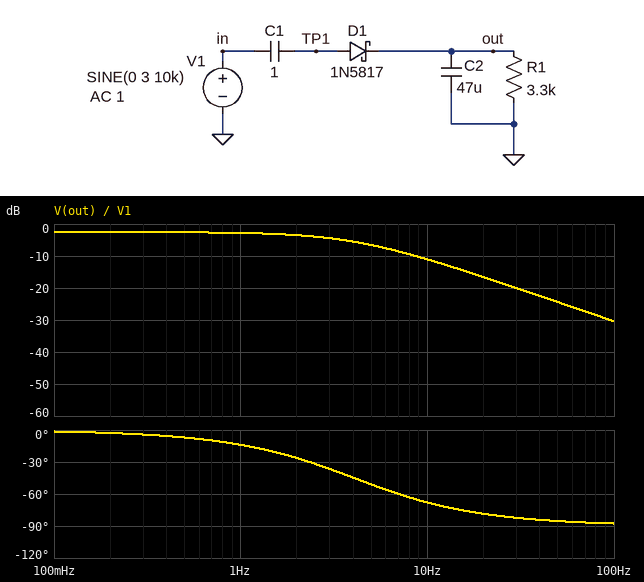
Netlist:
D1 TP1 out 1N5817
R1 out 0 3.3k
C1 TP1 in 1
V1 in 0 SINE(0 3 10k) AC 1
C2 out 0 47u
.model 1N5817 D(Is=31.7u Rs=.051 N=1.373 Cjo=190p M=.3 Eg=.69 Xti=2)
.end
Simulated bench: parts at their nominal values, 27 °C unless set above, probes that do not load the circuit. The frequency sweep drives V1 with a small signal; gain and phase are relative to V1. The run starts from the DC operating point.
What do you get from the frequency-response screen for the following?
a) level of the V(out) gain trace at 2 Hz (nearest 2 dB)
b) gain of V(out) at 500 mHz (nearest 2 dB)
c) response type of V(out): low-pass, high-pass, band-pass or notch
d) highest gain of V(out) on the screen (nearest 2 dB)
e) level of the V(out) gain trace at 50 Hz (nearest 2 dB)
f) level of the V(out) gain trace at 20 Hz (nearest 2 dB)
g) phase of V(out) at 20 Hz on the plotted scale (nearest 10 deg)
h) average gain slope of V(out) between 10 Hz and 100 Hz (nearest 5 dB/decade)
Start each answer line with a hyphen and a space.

- -4 dB
- -2 dB
- low-pass
- -2 dB
- -24 dB
- -16 dB
- -80 deg
- -20 dB/decade
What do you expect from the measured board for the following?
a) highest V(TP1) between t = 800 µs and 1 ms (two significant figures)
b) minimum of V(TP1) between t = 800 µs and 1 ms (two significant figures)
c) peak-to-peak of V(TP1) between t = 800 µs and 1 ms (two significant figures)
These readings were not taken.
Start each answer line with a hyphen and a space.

- 3.0 V
- -3.0 V
- 6.0 V
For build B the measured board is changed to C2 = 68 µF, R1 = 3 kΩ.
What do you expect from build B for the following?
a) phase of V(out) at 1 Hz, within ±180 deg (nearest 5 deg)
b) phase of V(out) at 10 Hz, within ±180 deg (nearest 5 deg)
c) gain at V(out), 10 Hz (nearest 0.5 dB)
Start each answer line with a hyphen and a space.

- -20 deg
- -75 deg
- -14.0 dB
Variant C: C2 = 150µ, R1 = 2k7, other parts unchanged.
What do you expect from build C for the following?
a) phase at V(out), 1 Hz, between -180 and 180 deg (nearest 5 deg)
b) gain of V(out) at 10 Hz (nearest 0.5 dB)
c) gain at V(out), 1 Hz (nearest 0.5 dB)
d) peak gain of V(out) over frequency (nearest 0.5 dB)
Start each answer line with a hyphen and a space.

- -35 deg
- -20.5 dB
- -5.0 dB
- -3.0 dB
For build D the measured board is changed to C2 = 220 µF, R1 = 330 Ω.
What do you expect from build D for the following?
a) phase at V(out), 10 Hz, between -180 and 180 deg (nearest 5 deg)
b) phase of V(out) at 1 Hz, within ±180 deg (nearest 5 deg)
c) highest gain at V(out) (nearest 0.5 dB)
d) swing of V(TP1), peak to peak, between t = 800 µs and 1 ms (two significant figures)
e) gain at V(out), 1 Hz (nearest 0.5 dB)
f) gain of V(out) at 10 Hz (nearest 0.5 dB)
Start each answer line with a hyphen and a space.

- -75 deg
- -20 deg
- -13.0 dB
- 6.0 V
- -13.5 dB
- -24.0 dB
